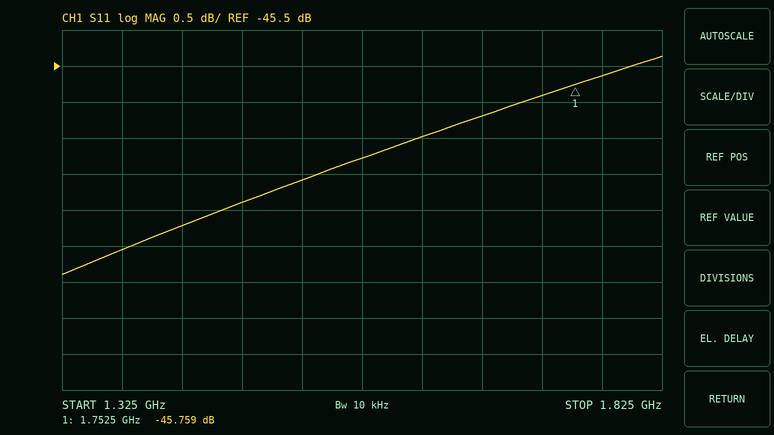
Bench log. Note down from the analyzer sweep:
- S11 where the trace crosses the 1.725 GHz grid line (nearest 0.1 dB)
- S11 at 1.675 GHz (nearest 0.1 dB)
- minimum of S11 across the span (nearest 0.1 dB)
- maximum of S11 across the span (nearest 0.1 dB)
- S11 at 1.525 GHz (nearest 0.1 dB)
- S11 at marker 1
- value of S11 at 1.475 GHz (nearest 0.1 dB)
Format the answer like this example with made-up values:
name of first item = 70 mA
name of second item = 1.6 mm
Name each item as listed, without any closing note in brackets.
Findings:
S11 where the trace crosses the 1.725 GHz grid line = -45.9 dB
S11 at 1.675 GHz = -46.2 dB
minimum of S11 across the span = -48.4 dB
maximum of S11 across the span = -45.4 dB
S11 at 1.525 GHz = -47.1 dB
S11 at marker 1 = -45.759 dB
value of S11 at 1.475 GHz = -47.4 dB
